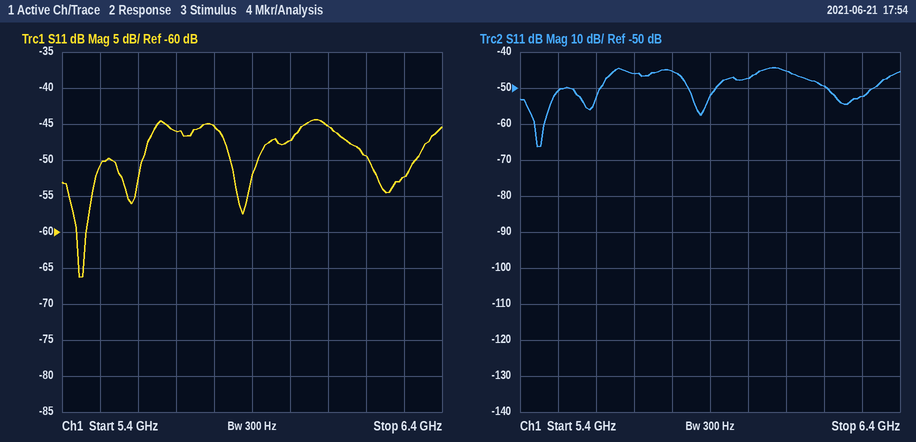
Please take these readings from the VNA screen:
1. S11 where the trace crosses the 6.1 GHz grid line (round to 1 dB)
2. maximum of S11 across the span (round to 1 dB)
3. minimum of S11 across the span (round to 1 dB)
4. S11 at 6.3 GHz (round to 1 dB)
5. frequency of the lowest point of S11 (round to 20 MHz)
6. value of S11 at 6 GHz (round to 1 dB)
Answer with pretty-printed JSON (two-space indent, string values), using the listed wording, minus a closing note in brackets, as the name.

{
  "S11 where the trace crosses the 6.1 GHz grid line": "-45 dB",
  "maximum of S11 across the span": "-44 dB",
  "minimum of S11 across the span": "-66 dB",
  "S11 at 6.3 GHz": "-52 dB",
  "frequency of the lowest point of S11": "5.44 GHz",
  "value of S11 at 6 GHz": "-47 dB"
}
